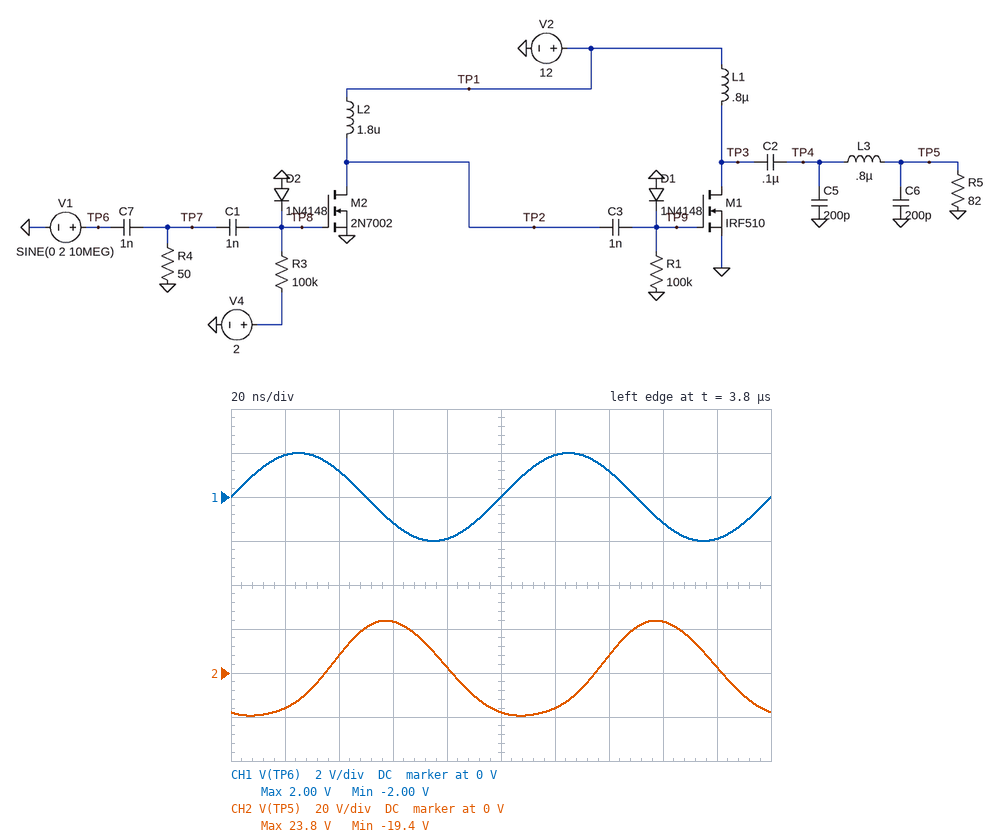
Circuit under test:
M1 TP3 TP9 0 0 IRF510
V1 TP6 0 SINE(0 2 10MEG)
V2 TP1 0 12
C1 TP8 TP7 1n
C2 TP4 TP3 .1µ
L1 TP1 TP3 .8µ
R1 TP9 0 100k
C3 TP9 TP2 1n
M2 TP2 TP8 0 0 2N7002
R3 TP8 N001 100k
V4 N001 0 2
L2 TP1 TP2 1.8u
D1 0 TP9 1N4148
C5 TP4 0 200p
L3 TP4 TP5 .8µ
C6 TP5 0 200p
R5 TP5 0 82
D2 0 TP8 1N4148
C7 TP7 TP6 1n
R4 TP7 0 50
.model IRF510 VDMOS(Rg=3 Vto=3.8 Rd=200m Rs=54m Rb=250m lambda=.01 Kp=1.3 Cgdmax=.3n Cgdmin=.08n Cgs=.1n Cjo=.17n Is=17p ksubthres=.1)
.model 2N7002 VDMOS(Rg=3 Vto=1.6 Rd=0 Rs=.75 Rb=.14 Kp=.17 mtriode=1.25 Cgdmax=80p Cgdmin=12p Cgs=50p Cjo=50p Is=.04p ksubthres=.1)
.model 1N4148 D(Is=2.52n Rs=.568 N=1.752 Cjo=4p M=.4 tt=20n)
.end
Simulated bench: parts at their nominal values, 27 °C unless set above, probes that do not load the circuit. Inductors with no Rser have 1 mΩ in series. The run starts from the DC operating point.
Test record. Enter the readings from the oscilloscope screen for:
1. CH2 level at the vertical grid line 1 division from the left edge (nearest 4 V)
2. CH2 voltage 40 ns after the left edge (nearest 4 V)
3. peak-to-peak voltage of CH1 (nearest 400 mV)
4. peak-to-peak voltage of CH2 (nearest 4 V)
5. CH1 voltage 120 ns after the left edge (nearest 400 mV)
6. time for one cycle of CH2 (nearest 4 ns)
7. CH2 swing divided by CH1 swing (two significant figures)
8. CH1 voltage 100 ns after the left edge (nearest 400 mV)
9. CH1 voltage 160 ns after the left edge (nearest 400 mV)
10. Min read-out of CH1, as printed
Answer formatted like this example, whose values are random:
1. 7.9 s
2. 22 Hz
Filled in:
1. -16 V
2. 8 V
3. 4.0 V
4. 44 V
5. 2.0 V
6. 100 ns
7. 11
8. 0 V
9. -1.2 V
10. -2.00 V
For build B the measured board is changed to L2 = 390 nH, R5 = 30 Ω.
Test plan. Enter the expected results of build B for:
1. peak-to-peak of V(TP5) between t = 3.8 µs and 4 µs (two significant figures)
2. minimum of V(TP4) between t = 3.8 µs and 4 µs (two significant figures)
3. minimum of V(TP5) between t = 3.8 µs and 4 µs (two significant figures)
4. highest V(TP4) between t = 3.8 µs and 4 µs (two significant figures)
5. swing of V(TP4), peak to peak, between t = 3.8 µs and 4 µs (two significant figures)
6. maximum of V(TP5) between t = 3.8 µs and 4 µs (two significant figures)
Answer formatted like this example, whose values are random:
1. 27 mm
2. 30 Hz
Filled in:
1. 24 V
2. -13 V
3. -10 V
4. 30 V
5. 43 V
6. 14 V
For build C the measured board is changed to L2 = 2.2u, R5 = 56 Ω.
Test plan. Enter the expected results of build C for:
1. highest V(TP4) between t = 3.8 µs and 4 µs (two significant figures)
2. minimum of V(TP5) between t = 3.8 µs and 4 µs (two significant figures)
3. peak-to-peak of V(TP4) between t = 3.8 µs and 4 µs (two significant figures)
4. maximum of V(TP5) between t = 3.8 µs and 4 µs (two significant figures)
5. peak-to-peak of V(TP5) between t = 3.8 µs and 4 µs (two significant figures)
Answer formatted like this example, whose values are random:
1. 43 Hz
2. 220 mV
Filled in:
1. 23 V
2. -14 V
3. 35 V
4. 19 V
5. 33 V
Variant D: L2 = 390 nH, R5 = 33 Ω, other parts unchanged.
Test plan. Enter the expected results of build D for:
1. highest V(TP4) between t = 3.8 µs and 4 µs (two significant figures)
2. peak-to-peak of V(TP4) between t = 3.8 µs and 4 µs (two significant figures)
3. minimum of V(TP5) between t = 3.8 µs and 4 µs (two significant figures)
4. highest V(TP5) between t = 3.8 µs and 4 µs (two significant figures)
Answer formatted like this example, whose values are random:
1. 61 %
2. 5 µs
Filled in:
1. 30 V
2. 42 V
3. -11 V
4. 15 V
